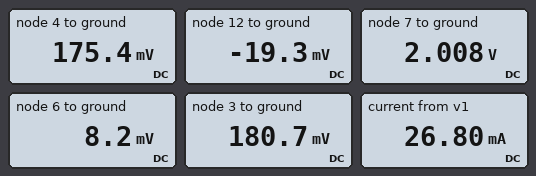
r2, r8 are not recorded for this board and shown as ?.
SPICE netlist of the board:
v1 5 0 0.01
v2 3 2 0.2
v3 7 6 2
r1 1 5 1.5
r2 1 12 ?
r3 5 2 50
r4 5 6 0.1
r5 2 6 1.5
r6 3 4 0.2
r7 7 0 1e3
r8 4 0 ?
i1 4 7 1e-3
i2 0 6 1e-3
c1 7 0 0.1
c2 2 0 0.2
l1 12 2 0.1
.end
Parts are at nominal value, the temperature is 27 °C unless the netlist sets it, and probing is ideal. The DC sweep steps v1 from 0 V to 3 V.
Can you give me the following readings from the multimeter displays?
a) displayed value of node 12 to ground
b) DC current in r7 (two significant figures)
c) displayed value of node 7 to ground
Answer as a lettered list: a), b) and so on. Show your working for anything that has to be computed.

a) -19.3 mV
b) (2.008 V) / 1 kΩ = 2.0 mA
c) 2.008 V
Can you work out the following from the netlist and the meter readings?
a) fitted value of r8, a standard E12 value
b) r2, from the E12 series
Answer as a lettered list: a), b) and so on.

a) 6.8 Ω
b) 2.2 Ω
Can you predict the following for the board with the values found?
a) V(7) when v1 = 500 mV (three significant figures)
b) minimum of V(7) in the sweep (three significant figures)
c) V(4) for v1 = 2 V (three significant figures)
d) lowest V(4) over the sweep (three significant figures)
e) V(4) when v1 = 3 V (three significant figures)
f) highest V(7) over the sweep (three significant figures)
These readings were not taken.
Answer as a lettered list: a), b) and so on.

a) 2.49 V
b) 2.00 V
c) 1.85 V
d) 167 mV
e) 2.69 V
f) 4.97 V
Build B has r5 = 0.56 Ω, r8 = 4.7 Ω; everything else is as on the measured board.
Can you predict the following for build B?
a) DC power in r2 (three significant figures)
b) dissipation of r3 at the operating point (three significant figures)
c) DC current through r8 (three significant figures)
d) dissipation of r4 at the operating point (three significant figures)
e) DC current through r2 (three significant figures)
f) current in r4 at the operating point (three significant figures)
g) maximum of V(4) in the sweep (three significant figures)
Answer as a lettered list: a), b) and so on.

a) 76.4 µW
b) 9.51 µW
c) 38.4 mA
d) 109 µW
e) 5.89 mA
f) 33.0 mA
g) 2.76 V
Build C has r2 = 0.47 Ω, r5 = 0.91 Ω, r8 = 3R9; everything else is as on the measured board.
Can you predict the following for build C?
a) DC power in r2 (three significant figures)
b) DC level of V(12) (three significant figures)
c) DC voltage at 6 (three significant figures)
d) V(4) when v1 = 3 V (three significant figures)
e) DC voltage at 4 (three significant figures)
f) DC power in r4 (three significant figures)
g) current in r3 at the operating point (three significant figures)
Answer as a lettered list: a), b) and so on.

a) 106 µW
b) -19.6 mV
c) 7.07 mV
d) 2.62 V
e) 171 mV
f) 86.0 µW
g) 592 µA
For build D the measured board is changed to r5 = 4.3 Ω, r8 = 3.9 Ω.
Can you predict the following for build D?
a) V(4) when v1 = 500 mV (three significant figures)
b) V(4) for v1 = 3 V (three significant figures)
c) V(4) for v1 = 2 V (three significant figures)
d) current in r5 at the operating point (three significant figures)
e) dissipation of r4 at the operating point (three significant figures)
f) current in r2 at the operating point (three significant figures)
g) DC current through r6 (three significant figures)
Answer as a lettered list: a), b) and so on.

a) 451 mV
b) 2.07 V
c) 1.42 V
d) 15.6 mA
e) 24.3 µW
f) 18.5 mA
g) 35.5 mA
